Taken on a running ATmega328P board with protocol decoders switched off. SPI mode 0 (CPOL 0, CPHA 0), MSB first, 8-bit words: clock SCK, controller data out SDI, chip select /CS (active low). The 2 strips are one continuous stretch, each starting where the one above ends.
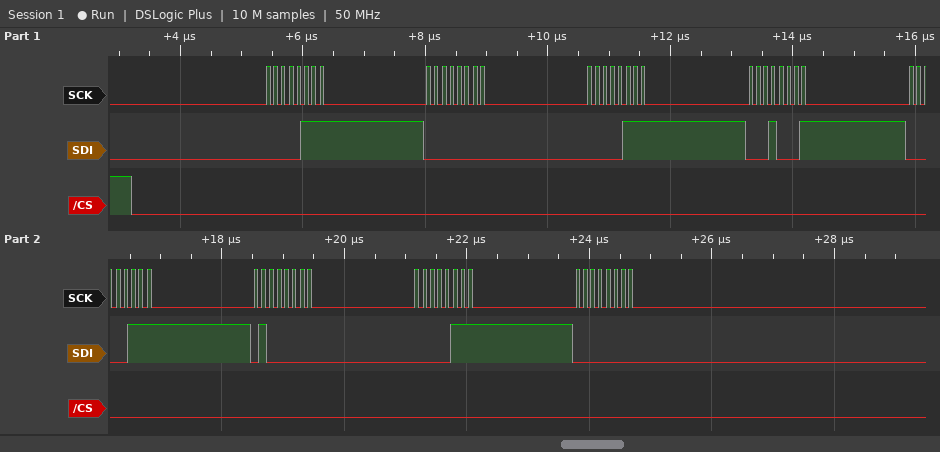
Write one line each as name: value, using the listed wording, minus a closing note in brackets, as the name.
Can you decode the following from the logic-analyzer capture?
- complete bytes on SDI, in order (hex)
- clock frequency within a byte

complete bytes on SDI, in order: 07 00 07 11 07 40 07 00
clock frequency within a byte: 8 MHz
